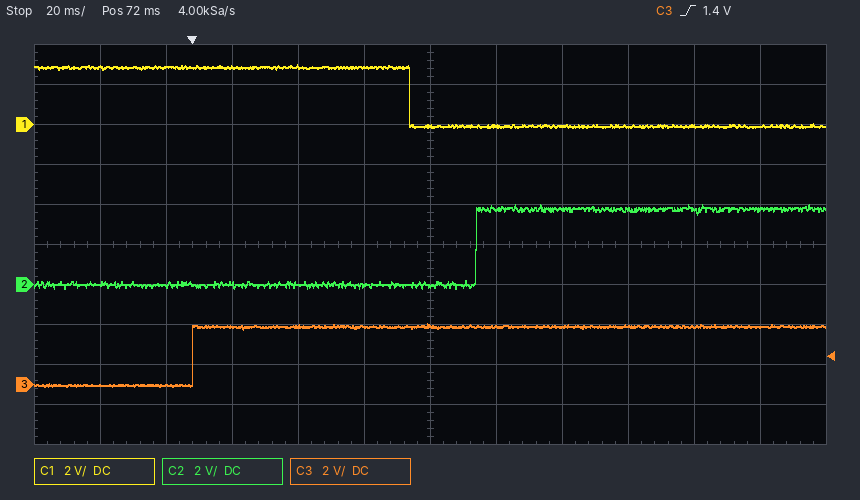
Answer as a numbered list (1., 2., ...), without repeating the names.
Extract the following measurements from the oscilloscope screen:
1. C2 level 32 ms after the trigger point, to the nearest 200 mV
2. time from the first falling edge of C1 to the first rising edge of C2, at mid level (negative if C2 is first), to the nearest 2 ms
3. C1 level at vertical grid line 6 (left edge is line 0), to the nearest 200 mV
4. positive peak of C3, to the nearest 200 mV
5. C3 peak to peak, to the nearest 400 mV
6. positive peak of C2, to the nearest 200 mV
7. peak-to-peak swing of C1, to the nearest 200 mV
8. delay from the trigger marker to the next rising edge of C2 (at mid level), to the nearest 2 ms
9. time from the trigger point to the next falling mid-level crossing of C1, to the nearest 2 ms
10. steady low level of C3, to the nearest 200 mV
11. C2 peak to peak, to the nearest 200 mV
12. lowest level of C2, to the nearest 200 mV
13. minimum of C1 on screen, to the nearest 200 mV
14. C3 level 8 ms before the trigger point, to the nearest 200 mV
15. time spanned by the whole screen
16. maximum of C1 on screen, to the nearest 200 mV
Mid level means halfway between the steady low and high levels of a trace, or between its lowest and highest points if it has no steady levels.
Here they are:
1. 0.0 V
2. +20 ms
3. 0.0 V
4. 3.0 V
5. 3.2 V
6. 4.0 V
7. 3.2 V
8. 86 ms
9. 66 ms
10. 0.0 V
11. 4.2 V
12. -200 mV
13. -200 mV
14. 0.0 V
15. 240 ms
16. 3.0 V
